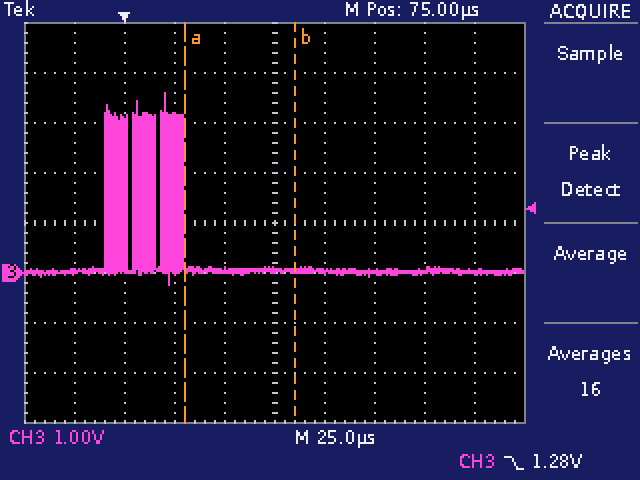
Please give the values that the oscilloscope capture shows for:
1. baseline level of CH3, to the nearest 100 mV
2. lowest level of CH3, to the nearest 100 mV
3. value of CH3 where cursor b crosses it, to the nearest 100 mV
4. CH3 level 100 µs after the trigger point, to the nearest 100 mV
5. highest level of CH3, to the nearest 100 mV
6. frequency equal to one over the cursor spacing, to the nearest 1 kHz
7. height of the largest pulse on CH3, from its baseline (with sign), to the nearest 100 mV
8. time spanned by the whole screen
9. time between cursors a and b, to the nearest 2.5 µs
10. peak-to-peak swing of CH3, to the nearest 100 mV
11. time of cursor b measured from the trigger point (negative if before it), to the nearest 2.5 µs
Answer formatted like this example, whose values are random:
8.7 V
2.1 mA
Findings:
0.0 V
-200 mV
100 mV
0.0 V
3.6 V
18 kHz
+3.6 V
250 µs
55.0 µs
3.8 V
+85.0 µs
